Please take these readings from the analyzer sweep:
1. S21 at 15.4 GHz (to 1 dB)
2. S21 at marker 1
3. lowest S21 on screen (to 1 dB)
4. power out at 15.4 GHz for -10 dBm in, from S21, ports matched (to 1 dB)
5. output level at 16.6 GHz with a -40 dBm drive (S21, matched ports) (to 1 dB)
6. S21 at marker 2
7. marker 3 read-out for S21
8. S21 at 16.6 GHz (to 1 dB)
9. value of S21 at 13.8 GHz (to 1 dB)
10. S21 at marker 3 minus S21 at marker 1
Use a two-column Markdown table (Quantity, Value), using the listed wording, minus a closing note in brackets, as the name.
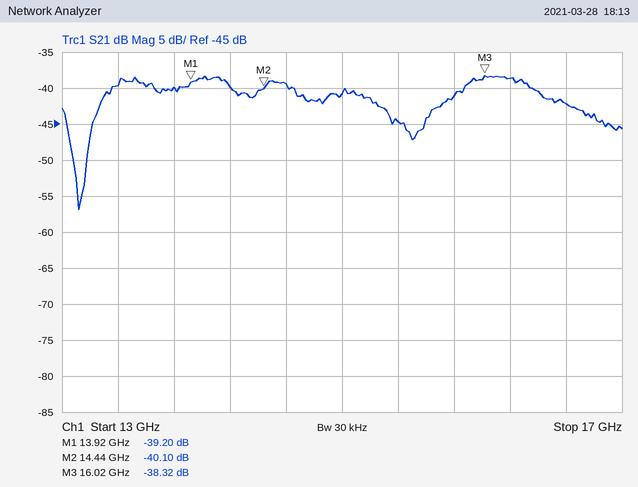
| Quantity | Value |
|---|---|
| S21 at 15.4 GHz | -45 dB |
| S21 at marker 1 | -39.20 dB |
| lowest S21 on screen | -57 dB |
| power out at 15.4 GHz for -10 dBm in, from S21, ports matched | -55 dBm |
| output level at 16.6 GHz with a -40 dBm drive (S21, matched ports) | -82 dBm |
| S21 at marker 2 | -40.10 dB |
| marker 3 read-out for S21 | -38.32 dB |
| S21 at 16.6 GHz | -42 dB |
| value of S21 at 13.8 GHz | -40 dB |
| S21 at marker 3 minus S21 at marker 1 | 0.88 dB |
